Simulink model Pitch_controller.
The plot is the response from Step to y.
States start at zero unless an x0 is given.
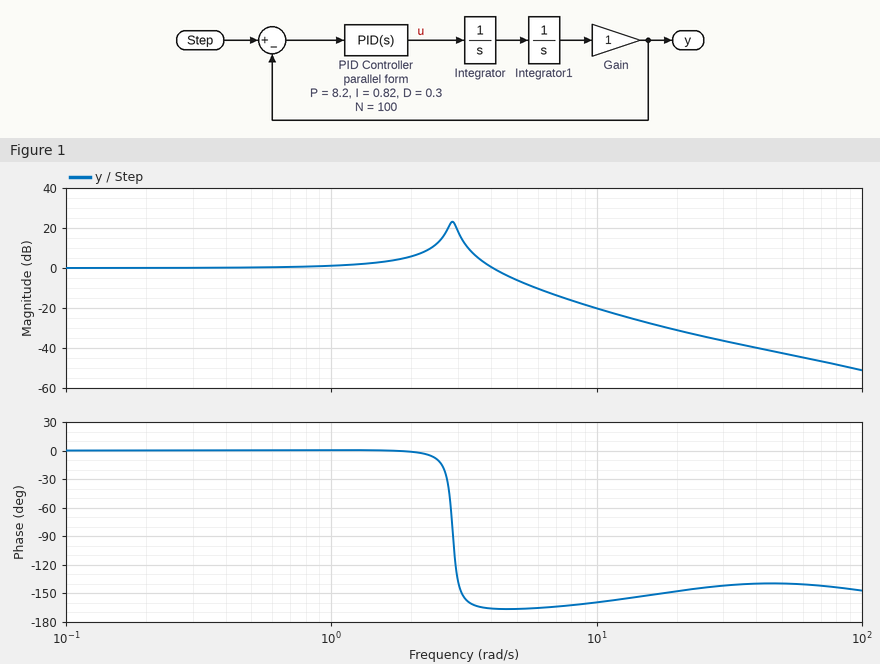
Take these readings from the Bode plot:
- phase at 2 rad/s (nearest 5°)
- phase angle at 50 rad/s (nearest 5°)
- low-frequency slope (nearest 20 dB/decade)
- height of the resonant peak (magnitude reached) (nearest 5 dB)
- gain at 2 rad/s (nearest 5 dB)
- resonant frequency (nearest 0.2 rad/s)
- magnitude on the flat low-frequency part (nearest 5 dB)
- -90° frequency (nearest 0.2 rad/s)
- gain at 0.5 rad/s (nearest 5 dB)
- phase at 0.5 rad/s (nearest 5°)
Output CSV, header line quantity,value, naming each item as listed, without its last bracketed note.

quantity,value
phase at 2 rad/s,0°
phase angle at 50 rad/s,-140°
low-frequency slope,0 dB/decade
height of the resonant peak (magnitude reached),25 dB
gain at 2 rad/s,5 dB
resonant frequency,2.8 rad/s
magnitude on the flat low-frequency part,0 dB
-90° frequency,2.8 rad/s
gain at 0.5 rad/s,0 dB
phase at 0.5 rad/s,0°
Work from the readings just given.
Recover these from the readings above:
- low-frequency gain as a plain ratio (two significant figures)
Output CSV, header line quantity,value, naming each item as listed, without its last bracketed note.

quantity,value
low-frequency gain as a plain ratio,1.0
